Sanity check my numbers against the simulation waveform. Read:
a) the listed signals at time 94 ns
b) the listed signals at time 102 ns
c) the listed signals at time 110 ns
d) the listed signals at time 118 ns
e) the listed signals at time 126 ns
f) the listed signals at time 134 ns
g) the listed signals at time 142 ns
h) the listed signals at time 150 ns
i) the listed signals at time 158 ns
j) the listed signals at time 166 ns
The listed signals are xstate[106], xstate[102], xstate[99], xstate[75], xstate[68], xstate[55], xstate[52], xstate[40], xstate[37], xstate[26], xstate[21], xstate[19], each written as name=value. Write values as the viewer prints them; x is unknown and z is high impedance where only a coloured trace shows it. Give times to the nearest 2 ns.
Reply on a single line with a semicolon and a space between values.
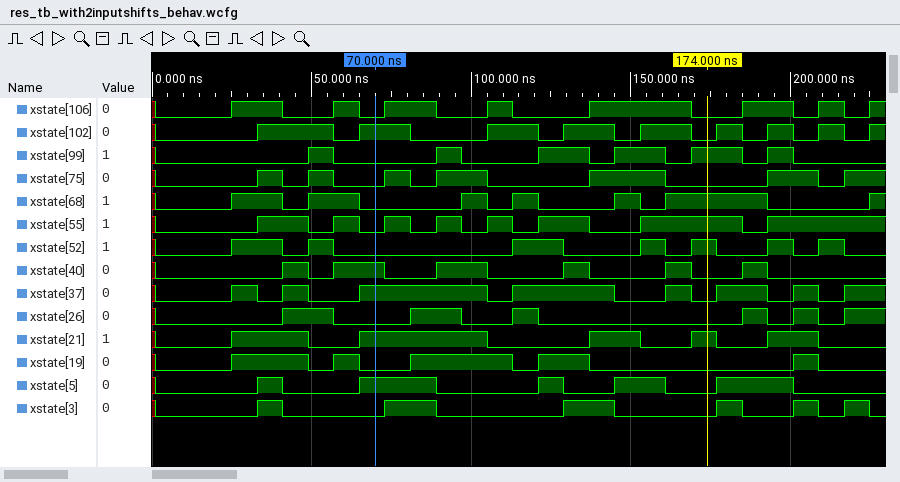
xstate[106]=0, xstate[102]=0, xstate[99]=1, xstate[75]=1, xstate[68]=0, xstate[55]=1, xstate[52]=0, xstate[40]=1, xstate[37]=1, xstate[26]=1, xstate[21]=1, xstate[19]=1; xstate[106]=0, xstate[102]=0, xstate[99]=0, xstate[75]=1, xstate[68]=1, xstate[55]=0, xstate[52]=0, xstate[40]=1, xstate[37]=1, xstate[26]=0, xstate[21]=1, xstate[19]=1; xstate[106]=1, xstate[102]=1, xstate[99]=0, xstate[75]=0, xstate[68]=0, xstate[55]=1, xstate[52]=0, xstate[40]=0, xstate[37]=0, xstate[26]=0, xstate[21]=0, xstate[19]=1; xstate[106]=0, xstate[102]=1, xstate[99]=0, xstate[75]=0, xstate[68]=1, xstate[55]=0, xstate[52]=1, xstate[40]=0, xstate[37]=1, xstate[26]=1, xstate[21]=0, xstate[19]=0; xstate[106]=0, xstate[102]=0, xstate[99]=1, xstate[75]=0, xstate[68]=0, xstate[55]=1, xstate[52]=1, xstate[40]=0, xstate[37]=1, xstate[26]=0, xstate[21]=0, xstate[19]=1; xstate[106]=0, xstate[102]=1, xstate[99]=1, xstate[75]=0, xstate[68]=0, xstate[55]=1, xstate[52]=0, xstate[40]=1, xstate[37]=1, xstate[26]=0, xstate[21]=0, xstate[19]=1; xstate[106]=1, xstate[102]=1, xstate[99]=0, xstate[75]=1, xstate[68]=0, xstate[55]=0, xstate[52]=0, xstate[40]=0, xstate[37]=1, xstate[26]=0, xstate[21]=1, xstate[19]=0; xstate[106]=1, xstate[102]=0, xstate[99]=1, xstate[75]=1, xstate[68]=1, xstate[55]=0, xstate[52]=0, xstate[40]=0, xstate[37]=0, xstate[26]=0, xstate[21]=1, xstate[19]=0; xstate[106]=1, xstate[102]=1, xstate[99]=1, xstate[75]=1, xstate[68]=0, xstate[55]=1, xstate[52]=1, xstate[40]=0, xstate[37]=0, xstate[26]=0, xstate[21]=0, xstate[19]=0; xstate[106]=1, xstate[102]=1, xstate[99]=0, xstate[75]=0, xstate[68]=1, xstate[55]=1, xstate[52]=0, xstate[40]=1, xstate[37]=1, xstate[26]=0, xstate[21]=0, xstate[19]=0
